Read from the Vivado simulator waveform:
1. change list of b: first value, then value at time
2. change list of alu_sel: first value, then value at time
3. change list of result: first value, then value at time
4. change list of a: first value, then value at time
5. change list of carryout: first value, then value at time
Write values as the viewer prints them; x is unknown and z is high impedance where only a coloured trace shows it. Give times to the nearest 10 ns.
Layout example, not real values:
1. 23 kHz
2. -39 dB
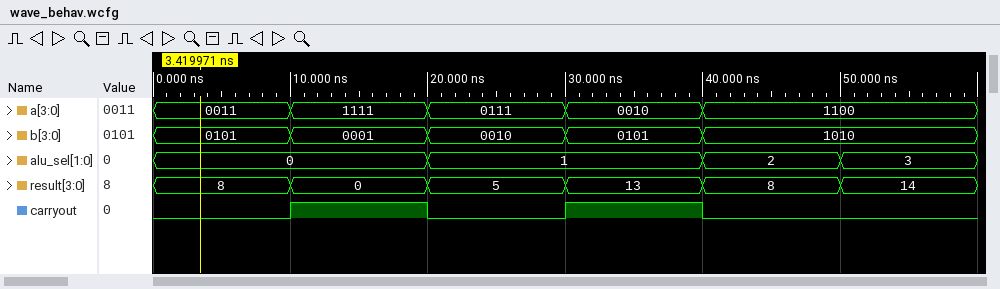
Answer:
1. 0101, 0001 at 10 ns, 0010 at 20 ns, 0101 at 30 ns, 1010 at 40 ns
2. 0, 1 at 20 ns, 2 at 40 ns, 3 at 50 ns
3. 8, 0 at 10 ns, 5 at 20 ns, 13 at 30 ns, 8 at 40 ns, 14 at 50 ns
4. 0011, 1111 at 10 ns, 0111 at 20 ns, 0010 at 30 ns, 1100 at 40 ns
5. 0, 1 at 10 ns, 0 at 20 ns, 1 at 30 ns, 0 at 40 ns
